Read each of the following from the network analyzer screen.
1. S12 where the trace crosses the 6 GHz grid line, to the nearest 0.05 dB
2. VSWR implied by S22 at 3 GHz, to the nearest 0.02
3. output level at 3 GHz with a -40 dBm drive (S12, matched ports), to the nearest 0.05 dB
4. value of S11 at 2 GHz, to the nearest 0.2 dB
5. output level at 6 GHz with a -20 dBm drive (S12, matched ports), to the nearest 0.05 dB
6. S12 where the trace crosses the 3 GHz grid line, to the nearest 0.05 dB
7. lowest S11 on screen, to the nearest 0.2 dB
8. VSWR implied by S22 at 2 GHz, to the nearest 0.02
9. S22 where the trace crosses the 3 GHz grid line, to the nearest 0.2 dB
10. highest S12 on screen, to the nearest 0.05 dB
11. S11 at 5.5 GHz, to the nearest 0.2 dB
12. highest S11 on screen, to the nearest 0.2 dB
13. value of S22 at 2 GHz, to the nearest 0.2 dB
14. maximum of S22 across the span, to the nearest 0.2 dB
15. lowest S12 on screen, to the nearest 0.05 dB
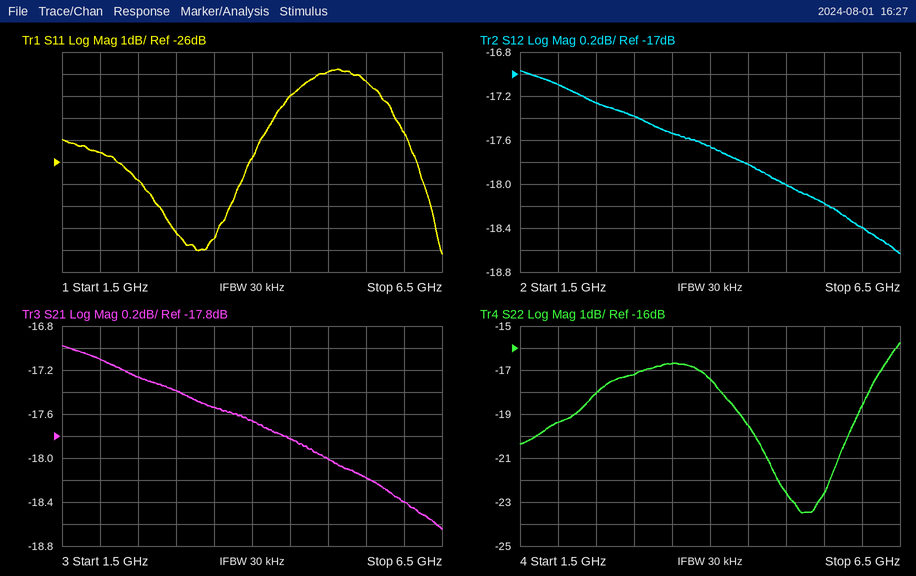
-18.40 dB
1.32
-57.40 dBm
-25.6 dB
-38.40 dBm
-17.40 dB
-30.2 dB
1.24
-17.2 dB
-16.95 dB
-22.4 dB
-21.8 dB
-19.4 dB
-15.8 dB
-18.65 dB
